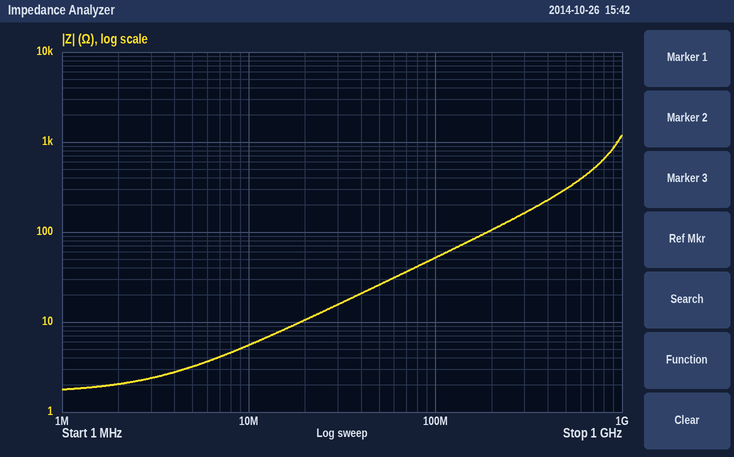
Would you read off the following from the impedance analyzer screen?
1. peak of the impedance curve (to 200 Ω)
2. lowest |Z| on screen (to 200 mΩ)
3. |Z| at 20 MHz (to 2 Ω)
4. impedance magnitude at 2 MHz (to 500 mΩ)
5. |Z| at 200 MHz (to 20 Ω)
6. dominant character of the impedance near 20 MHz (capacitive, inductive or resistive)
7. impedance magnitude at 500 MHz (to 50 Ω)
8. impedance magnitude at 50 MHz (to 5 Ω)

1.2 kΩ
1.8 Ω
10 Ω
2.0 Ω
100 Ω
inductive
300 Ω
25 Ω
